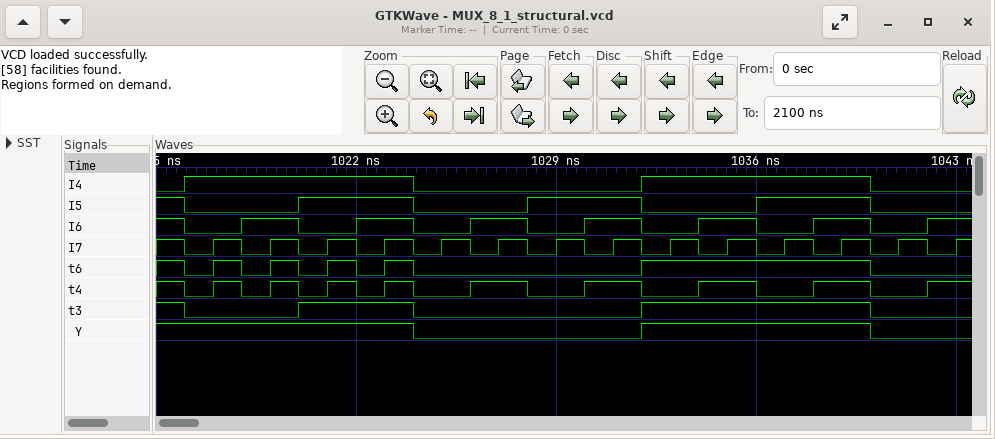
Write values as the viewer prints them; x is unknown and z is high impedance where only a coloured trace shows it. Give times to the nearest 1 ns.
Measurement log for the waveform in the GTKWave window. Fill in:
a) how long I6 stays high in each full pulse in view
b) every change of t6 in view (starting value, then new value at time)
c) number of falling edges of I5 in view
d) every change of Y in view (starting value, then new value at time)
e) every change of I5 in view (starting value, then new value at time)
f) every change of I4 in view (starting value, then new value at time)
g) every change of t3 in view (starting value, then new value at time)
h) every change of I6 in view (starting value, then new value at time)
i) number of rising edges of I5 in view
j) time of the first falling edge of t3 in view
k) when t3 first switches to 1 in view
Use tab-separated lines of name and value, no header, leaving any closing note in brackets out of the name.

how long I6 stays high in each full pulse in view	2 ns, 2 ns, 2 ns, 2 ns, 2 ns, 2 ns
every change of t6 in view	1, 0 at 1016 ns, 1 at 1017 ns, 0 at 1018 ns, 1 at 1019 ns, 0 at 1020 ns, 1 at 1021 ns, 0 at 1022 ns, 1 at 1023 ns, 0 at 1024 ns, 1 at 1032 ns, 0 at 1040 ns
number of falling edges of I5 in view	4
every change of Y in view	1, 0 at 1024 ns, 1 at 1032 ns, 0 at 1040 ns
every change of I5 in view	1, 0 at 1016 ns, 1 at 1020 ns, 0 at 1024 ns, 1 at 1028 ns, 0 at 1032 ns, 1 at 1036 ns, 0 at 1040 ns
every change of I4 in view	0, 1 at 1016 ns, 0 at 1024 ns, 1 at 1032 ns, 0 at 1040 ns
every change of t3 in view	1, 0 at 1016 ns, 1 at 1020 ns, 0 at 1024 ns, 1 at 1032 ns, 0 at 1040 ns
every change of I6 in view	1, 0 at 1016 ns, 1 at 1018 ns, 0 at 1020 ns, 1 at 1022 ns, 0 at 1024 ns, 1 at 1026 ns, 0 at 1028 ns, 1 at 1030 ns, 0 at 1032 ns, 1 at 1034 ns, 0 at 1036 ns, 1 at 1038 ns, 0 at 1040 ns, 1 at 1042 ns
number of rising edges of I5 in view	3
time of the first falling edge of t3 in view	1016 ns
when t3 first switches to 1 in view	1020 ns
